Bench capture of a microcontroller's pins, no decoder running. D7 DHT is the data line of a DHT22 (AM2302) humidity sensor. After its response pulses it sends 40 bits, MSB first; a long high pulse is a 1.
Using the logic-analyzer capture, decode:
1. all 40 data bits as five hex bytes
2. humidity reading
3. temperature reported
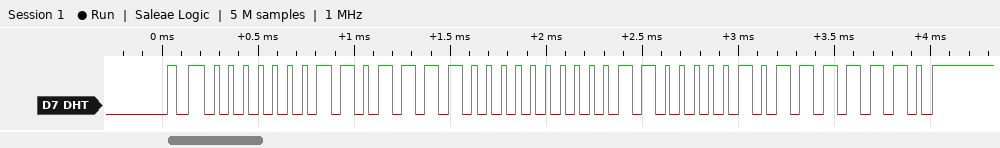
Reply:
01 BC 00 C1 7E
44.4 %
19.3 °C
